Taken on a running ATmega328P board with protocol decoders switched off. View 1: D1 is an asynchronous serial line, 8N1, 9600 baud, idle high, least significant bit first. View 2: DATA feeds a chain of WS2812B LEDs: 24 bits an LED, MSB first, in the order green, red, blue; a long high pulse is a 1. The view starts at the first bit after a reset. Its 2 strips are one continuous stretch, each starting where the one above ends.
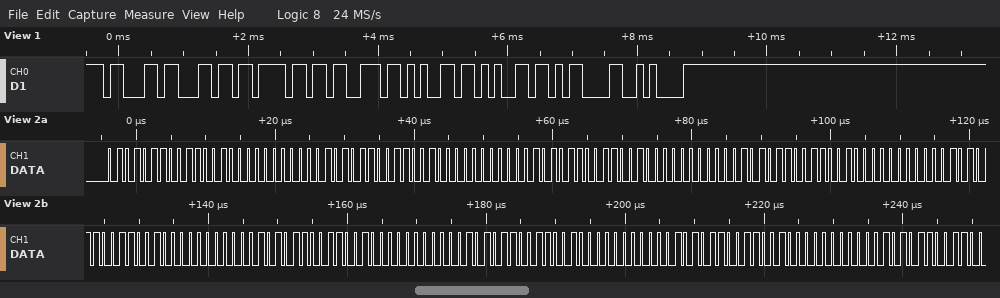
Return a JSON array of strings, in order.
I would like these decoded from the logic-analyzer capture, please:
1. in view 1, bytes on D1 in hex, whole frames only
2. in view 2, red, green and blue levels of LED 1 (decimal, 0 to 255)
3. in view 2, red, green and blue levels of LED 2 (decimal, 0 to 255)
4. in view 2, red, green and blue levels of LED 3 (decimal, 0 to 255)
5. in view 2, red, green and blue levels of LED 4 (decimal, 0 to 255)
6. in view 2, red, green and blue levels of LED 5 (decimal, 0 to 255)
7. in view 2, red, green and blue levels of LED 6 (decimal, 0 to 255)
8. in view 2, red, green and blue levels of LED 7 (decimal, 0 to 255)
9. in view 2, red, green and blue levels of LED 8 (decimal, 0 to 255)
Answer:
["63 6C 6F 73 65 65 0D 0A", "100, 86, 0", "100, 86, 0", "100, 86, 0", "100, 86, 0", "100, 86, 0", "100, 86, 0", "100, 86, 0", "100, 86, 0"]
